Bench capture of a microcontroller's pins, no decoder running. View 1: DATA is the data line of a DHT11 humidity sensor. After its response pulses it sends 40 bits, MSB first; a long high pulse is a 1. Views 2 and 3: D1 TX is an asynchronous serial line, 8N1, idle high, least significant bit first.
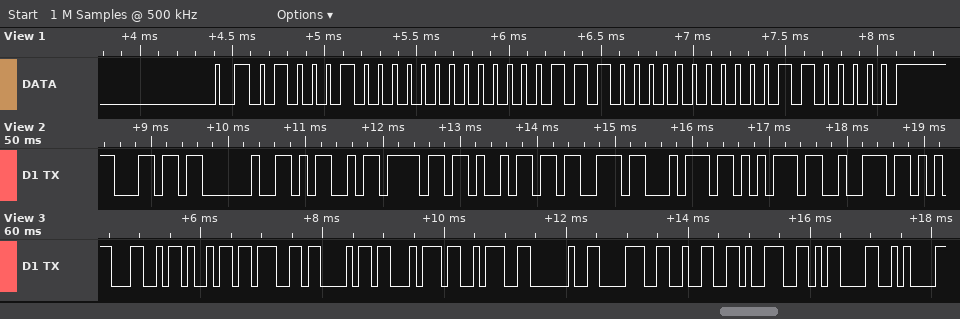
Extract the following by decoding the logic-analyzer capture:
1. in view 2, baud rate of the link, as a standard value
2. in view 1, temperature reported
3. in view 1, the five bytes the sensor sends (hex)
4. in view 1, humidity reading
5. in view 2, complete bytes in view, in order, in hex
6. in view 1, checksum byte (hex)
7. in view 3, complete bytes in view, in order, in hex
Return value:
9600 baud
28.0 °C
44 00 1C 00 60
68 %
6C 20 4D 6F 69 73 74 75 72
0x60
4C 69 67 68 74 3A 20 38 32 39 0D 0A
